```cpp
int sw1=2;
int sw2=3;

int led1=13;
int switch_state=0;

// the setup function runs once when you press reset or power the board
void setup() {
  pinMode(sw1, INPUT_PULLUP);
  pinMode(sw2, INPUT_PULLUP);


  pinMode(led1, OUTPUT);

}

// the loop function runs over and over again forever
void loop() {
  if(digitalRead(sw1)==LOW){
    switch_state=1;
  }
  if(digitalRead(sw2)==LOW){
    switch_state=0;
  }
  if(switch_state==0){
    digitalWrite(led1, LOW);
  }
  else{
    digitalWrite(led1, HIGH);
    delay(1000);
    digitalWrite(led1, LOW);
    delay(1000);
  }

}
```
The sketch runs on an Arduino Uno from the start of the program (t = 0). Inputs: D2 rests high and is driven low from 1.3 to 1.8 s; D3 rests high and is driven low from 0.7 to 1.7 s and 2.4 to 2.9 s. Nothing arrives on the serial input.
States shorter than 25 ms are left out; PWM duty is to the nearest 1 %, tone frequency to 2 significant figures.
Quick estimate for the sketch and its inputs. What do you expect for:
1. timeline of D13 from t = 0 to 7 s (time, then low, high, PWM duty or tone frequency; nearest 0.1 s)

0 s low; 1.7 s high; 2.7 s low; 3.7 s high; 4.7 s low; 5.7 s high; 6.7 s low
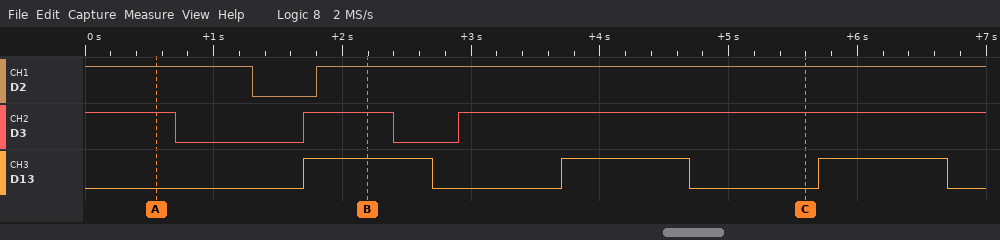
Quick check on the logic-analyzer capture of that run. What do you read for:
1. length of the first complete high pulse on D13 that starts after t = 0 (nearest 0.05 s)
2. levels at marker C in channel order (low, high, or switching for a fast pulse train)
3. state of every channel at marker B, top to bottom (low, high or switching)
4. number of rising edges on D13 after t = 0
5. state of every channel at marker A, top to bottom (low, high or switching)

1.00 s
D2 high, D3 high, D13 low
D2 high, D3 high, D13 high
3
D2 high, D3 high, D13 low
